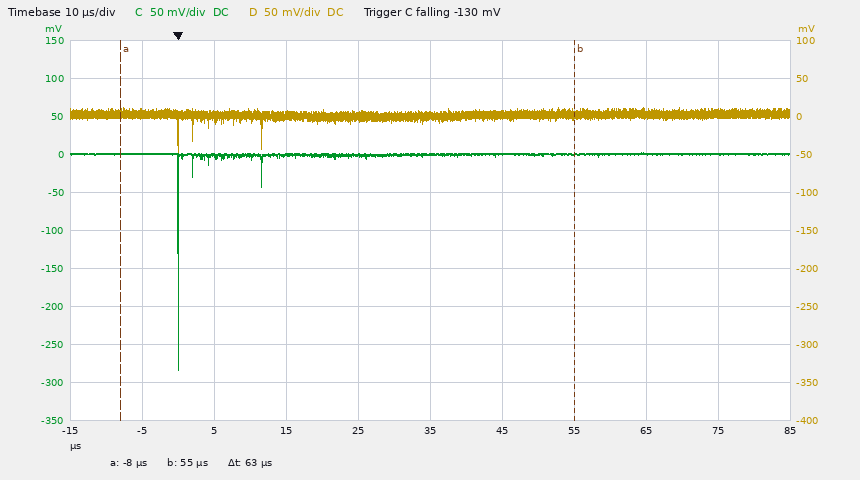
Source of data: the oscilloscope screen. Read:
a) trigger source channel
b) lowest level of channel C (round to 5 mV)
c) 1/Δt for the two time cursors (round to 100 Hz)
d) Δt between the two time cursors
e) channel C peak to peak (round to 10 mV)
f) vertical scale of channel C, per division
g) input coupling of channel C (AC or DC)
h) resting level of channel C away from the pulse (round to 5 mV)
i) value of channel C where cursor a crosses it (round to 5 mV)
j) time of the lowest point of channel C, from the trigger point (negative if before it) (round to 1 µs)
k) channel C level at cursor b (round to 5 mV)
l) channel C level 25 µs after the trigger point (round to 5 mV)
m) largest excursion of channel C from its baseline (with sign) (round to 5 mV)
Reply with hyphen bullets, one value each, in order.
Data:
- channel C
- -285 mV
- 15.9 kHz
- 63 µs
- 290 mV
- 50 mV
- DC
- 0 mV
- 0 mV
- 0 µs
- 0 mV
- 0 mV
- -285 mV
